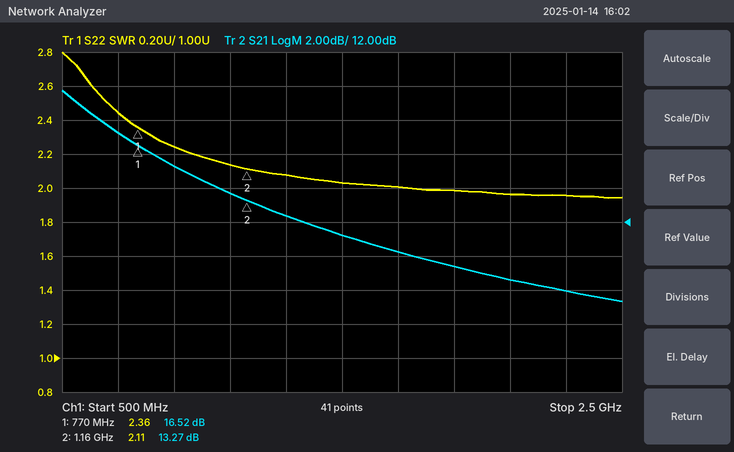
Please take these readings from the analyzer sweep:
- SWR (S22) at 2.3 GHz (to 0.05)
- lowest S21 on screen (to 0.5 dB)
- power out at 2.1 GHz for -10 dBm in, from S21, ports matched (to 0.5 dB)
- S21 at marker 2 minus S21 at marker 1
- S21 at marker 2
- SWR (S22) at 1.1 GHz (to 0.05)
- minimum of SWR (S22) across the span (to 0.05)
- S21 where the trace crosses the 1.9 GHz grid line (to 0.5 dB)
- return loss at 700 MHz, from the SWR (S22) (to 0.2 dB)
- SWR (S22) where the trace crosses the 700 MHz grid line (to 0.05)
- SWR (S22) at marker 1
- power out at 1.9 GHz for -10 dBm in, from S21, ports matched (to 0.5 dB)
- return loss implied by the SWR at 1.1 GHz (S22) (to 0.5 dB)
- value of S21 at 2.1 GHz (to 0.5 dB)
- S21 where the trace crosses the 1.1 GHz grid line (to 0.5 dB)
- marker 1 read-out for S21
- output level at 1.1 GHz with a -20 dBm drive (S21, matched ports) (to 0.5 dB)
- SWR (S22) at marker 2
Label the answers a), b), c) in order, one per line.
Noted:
a) 1.95
b) 7.5 dB
c) -1.5 dBm
d) -3.25 dB
e) 13.27 dB
f) 2.15
g) 1.95
h) 9.5 dB
i) 7.6 dB
j) 2.45
k) 2.36
l) -0.5 dBm
m) 9.0 dB
n) 8.5 dB
o) 13.5 dB
p) 16.52 dB
q) -6.5 dBm
r) 2.11
